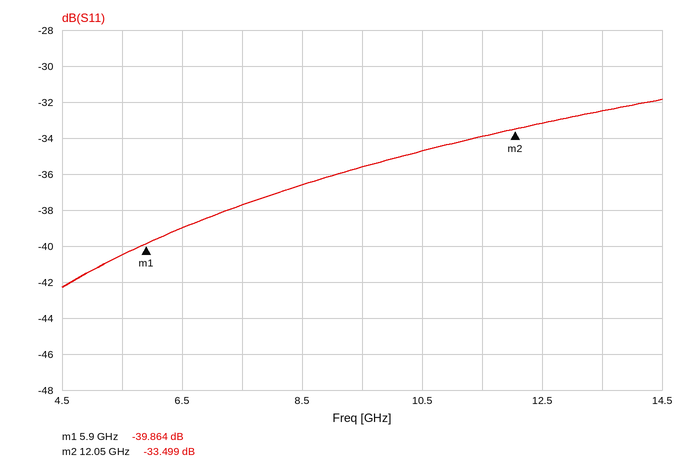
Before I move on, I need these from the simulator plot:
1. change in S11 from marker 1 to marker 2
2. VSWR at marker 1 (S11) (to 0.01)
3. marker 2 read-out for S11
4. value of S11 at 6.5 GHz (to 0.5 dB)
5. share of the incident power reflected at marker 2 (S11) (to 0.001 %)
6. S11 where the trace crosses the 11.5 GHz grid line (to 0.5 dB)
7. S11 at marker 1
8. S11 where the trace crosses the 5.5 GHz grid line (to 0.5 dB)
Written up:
6.365 dB
1.02
-33.499 dB
-39.0 dB
0.045 %
-34.0 dB
-39.864 dB
-40.5 dB
